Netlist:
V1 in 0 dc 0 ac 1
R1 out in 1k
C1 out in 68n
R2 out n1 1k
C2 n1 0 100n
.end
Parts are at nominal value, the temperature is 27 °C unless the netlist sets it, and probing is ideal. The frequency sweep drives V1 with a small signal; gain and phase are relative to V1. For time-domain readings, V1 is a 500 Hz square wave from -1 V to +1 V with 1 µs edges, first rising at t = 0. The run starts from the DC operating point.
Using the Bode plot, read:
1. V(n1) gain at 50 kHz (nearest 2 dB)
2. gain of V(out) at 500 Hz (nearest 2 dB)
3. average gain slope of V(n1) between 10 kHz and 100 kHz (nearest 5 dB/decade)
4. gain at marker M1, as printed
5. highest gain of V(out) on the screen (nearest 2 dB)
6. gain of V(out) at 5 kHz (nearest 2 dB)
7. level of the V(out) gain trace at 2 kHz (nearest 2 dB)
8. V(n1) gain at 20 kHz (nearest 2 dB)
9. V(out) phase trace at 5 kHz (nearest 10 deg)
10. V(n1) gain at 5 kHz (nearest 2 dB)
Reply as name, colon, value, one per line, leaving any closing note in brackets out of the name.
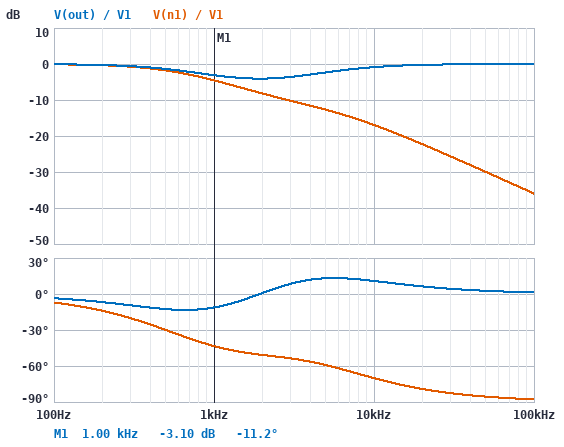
V(n1) gain at 50 kHz: -30 dB
gain of V(out) at 500 Hz: -2 dB
average gain slope of V(n1) between 10 kHz and 100 kHz: -20 dB/decade
gain at marker M1, as printed: -3.10 dB
highest gain of V(out) on the screen: 0 dB
gain of V(out) at 5 kHz: -2 dB
level of the V(out) gain trace at 2 kHz: -4 dB
V(n1) gain at 20 kHz: -22 dB
V(out) phase trace at 5 kHz: 10 deg
V(n1) gain at 5 kHz: -12 dB
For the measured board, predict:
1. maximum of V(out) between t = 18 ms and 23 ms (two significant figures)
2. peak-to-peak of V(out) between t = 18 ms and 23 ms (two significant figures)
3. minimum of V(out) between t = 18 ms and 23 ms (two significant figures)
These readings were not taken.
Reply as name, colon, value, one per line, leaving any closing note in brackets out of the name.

maximum of V(out) between t = 18 ms and 23 ms: 1.0 V
peak-to-peak of V(out) between t = 18 ms and 23 ms: 2.0 V
minimum of V(out) between t = 18 ms and 23 ms: -1.0 V
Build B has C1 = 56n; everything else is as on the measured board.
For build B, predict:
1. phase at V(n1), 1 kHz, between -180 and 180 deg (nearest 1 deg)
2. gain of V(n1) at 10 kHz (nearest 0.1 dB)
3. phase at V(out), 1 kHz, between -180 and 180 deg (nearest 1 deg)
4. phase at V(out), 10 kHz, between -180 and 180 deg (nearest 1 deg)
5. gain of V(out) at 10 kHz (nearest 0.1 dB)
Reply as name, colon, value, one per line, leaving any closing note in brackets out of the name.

phase at V(n1), 1 kHz, between -180 and 180 deg: -45 deg
gain of V(n1) at 10 kHz: -17.2 dB
phase at V(out), 1 kHz, between -180 and 180 deg: -13 deg
phase at V(out), 10 kHz, between -180 and 180 deg: 12 deg
gain of V(out) at 10 kHz: -1.1 dB
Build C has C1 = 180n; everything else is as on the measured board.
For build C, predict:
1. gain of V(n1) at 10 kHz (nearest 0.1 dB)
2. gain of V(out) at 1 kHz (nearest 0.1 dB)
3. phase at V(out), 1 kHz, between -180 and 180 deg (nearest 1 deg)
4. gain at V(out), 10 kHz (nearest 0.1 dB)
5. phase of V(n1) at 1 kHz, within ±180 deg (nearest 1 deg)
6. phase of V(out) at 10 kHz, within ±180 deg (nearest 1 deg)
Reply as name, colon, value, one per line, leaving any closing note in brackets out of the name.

gain of V(n1) at 10 kHz: -16.3 dB
gain of V(out) at 1 kHz: -2.6 dB
phase at V(out), 1 kHz, between -180 and 180 deg: -2 deg
gain at V(out), 10 kHz: -0.2 dB
phase of V(n1) at 1 kHz, within ±180 deg: -35 deg
phase of V(out) at 10 kHz, within ±180 deg: 5 deg
